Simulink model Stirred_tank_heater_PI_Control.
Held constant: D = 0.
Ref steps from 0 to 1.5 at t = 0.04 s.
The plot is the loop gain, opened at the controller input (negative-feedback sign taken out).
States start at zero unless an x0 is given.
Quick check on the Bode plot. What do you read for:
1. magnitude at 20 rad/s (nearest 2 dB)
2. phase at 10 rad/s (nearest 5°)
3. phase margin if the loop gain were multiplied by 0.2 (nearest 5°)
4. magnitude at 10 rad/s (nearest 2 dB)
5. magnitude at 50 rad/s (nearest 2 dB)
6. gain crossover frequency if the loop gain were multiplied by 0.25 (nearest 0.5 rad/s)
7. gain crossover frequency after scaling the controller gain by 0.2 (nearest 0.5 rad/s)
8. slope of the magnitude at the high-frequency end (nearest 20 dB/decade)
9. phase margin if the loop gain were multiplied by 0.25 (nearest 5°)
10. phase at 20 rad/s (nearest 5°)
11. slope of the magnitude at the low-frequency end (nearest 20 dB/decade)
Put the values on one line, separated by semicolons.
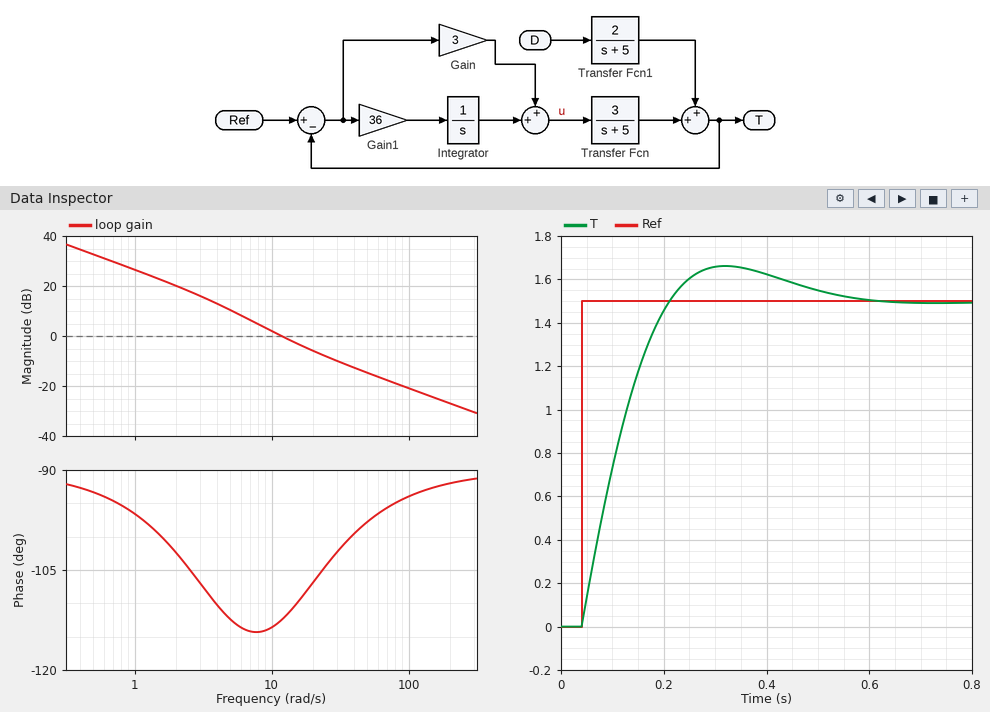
-6 dB; -115°; 70°; 2 dB; -14 dB; 4.5 rad/s; 3.5 rad/s; -20 dB/decade; 70°; -105°; -20 dB/decade
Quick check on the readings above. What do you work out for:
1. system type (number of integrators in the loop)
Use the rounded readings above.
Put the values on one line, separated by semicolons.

1
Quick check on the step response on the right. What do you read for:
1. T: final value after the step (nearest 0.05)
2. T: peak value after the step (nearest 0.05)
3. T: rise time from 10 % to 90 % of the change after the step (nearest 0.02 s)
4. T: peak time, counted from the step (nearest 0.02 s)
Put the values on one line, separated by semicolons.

1.50; 1.65; 0.12 s; 0.28 s
